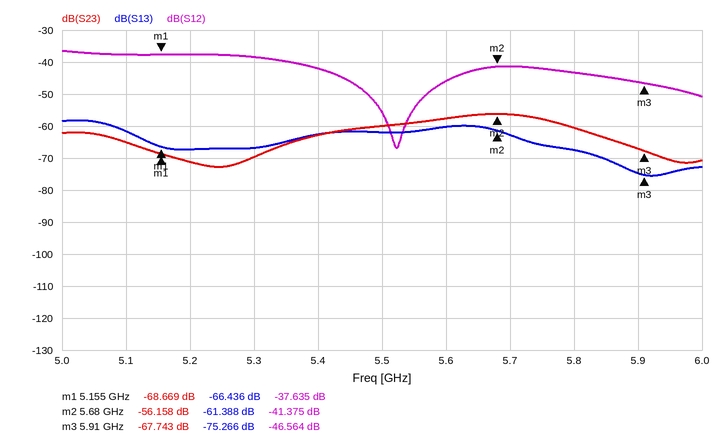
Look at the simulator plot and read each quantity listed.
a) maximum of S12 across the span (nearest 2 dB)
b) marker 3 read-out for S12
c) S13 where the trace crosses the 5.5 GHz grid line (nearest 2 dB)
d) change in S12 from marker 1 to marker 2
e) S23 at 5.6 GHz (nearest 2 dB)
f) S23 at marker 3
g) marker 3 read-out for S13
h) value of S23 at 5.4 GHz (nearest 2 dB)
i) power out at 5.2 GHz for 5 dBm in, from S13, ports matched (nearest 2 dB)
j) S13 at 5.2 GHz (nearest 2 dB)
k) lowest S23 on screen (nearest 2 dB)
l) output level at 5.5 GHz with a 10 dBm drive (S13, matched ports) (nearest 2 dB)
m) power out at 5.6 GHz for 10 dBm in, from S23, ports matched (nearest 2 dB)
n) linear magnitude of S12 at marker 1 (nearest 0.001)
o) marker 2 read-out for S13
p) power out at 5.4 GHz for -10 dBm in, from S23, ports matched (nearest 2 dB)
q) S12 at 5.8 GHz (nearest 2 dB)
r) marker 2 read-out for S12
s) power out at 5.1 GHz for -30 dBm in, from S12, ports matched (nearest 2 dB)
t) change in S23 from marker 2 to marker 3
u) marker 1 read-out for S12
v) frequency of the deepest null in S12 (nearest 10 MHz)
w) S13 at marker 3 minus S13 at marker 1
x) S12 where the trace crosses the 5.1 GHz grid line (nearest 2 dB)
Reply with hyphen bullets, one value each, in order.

- -36 dB
- -46.564 dB
- -62 dB
- -3.740 dB
- -58 dB
- -67.743 dB
- -75.266 dB
- -62 dB
- -62 dBm
- -68 dB
- -72 dB
- -52 dBm
- -48 dBm
- 0.013
- -61.388 dB
- -72 dBm
- -44 dB
- -41.375 dB
- -68 dBm
- -11.585 dB
- -37.635 dB
- 5.52 GHz
- -8.830 dB
- -38 dB
